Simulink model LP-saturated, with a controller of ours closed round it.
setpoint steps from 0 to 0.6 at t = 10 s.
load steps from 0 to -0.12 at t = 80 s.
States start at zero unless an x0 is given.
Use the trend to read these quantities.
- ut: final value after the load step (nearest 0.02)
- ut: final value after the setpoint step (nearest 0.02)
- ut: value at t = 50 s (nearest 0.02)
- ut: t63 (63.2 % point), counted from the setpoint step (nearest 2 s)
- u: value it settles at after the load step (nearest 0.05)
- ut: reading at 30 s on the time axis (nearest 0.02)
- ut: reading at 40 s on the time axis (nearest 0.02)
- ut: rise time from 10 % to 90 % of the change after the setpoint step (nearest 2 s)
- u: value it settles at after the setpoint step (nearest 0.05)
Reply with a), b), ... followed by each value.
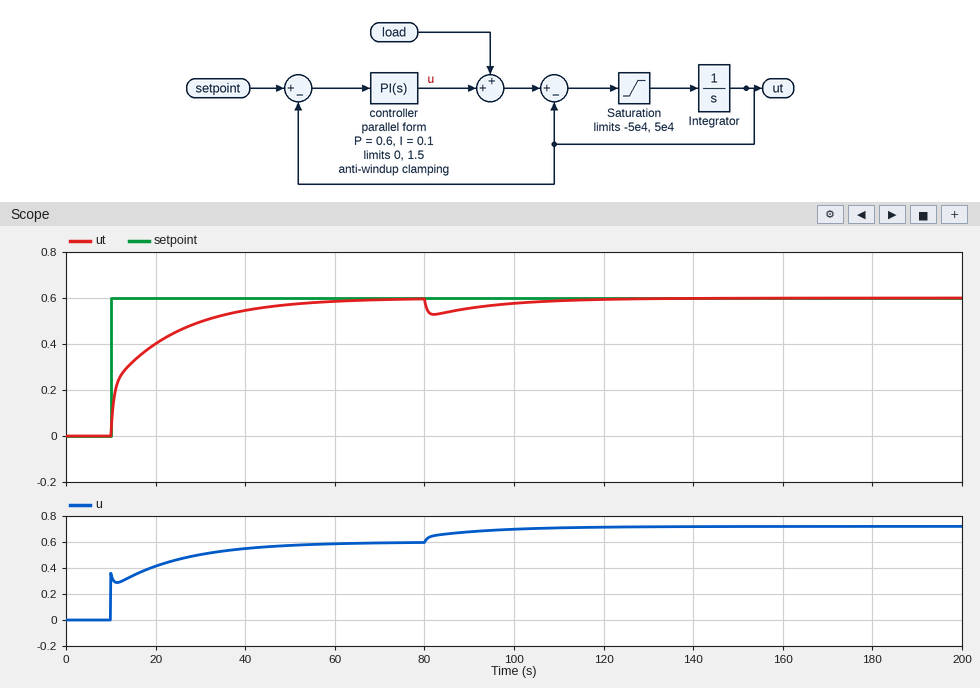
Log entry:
a) 0.60
b) 0.60
c) 0.58
d) 8 s
e) 0.70
f) 0.50
g) 0.54
h) 28 s
i) 0.60
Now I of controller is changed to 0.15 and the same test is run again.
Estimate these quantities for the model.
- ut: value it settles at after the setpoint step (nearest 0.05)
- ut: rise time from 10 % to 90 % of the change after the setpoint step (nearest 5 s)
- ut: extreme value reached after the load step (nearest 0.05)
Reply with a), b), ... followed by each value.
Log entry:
a) 0.60
b) 20 s
c) 0.55
